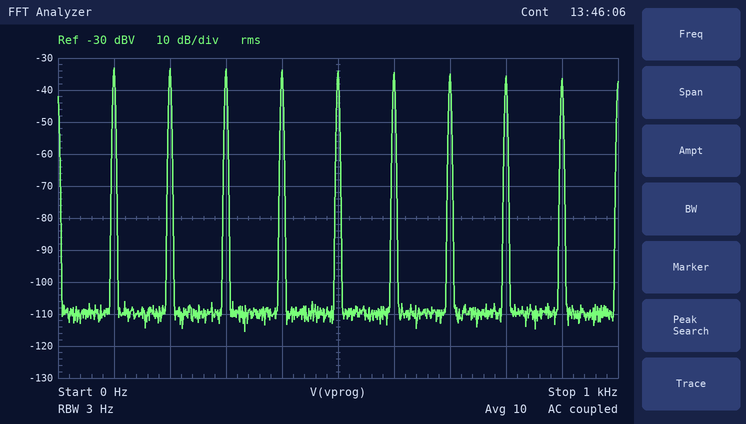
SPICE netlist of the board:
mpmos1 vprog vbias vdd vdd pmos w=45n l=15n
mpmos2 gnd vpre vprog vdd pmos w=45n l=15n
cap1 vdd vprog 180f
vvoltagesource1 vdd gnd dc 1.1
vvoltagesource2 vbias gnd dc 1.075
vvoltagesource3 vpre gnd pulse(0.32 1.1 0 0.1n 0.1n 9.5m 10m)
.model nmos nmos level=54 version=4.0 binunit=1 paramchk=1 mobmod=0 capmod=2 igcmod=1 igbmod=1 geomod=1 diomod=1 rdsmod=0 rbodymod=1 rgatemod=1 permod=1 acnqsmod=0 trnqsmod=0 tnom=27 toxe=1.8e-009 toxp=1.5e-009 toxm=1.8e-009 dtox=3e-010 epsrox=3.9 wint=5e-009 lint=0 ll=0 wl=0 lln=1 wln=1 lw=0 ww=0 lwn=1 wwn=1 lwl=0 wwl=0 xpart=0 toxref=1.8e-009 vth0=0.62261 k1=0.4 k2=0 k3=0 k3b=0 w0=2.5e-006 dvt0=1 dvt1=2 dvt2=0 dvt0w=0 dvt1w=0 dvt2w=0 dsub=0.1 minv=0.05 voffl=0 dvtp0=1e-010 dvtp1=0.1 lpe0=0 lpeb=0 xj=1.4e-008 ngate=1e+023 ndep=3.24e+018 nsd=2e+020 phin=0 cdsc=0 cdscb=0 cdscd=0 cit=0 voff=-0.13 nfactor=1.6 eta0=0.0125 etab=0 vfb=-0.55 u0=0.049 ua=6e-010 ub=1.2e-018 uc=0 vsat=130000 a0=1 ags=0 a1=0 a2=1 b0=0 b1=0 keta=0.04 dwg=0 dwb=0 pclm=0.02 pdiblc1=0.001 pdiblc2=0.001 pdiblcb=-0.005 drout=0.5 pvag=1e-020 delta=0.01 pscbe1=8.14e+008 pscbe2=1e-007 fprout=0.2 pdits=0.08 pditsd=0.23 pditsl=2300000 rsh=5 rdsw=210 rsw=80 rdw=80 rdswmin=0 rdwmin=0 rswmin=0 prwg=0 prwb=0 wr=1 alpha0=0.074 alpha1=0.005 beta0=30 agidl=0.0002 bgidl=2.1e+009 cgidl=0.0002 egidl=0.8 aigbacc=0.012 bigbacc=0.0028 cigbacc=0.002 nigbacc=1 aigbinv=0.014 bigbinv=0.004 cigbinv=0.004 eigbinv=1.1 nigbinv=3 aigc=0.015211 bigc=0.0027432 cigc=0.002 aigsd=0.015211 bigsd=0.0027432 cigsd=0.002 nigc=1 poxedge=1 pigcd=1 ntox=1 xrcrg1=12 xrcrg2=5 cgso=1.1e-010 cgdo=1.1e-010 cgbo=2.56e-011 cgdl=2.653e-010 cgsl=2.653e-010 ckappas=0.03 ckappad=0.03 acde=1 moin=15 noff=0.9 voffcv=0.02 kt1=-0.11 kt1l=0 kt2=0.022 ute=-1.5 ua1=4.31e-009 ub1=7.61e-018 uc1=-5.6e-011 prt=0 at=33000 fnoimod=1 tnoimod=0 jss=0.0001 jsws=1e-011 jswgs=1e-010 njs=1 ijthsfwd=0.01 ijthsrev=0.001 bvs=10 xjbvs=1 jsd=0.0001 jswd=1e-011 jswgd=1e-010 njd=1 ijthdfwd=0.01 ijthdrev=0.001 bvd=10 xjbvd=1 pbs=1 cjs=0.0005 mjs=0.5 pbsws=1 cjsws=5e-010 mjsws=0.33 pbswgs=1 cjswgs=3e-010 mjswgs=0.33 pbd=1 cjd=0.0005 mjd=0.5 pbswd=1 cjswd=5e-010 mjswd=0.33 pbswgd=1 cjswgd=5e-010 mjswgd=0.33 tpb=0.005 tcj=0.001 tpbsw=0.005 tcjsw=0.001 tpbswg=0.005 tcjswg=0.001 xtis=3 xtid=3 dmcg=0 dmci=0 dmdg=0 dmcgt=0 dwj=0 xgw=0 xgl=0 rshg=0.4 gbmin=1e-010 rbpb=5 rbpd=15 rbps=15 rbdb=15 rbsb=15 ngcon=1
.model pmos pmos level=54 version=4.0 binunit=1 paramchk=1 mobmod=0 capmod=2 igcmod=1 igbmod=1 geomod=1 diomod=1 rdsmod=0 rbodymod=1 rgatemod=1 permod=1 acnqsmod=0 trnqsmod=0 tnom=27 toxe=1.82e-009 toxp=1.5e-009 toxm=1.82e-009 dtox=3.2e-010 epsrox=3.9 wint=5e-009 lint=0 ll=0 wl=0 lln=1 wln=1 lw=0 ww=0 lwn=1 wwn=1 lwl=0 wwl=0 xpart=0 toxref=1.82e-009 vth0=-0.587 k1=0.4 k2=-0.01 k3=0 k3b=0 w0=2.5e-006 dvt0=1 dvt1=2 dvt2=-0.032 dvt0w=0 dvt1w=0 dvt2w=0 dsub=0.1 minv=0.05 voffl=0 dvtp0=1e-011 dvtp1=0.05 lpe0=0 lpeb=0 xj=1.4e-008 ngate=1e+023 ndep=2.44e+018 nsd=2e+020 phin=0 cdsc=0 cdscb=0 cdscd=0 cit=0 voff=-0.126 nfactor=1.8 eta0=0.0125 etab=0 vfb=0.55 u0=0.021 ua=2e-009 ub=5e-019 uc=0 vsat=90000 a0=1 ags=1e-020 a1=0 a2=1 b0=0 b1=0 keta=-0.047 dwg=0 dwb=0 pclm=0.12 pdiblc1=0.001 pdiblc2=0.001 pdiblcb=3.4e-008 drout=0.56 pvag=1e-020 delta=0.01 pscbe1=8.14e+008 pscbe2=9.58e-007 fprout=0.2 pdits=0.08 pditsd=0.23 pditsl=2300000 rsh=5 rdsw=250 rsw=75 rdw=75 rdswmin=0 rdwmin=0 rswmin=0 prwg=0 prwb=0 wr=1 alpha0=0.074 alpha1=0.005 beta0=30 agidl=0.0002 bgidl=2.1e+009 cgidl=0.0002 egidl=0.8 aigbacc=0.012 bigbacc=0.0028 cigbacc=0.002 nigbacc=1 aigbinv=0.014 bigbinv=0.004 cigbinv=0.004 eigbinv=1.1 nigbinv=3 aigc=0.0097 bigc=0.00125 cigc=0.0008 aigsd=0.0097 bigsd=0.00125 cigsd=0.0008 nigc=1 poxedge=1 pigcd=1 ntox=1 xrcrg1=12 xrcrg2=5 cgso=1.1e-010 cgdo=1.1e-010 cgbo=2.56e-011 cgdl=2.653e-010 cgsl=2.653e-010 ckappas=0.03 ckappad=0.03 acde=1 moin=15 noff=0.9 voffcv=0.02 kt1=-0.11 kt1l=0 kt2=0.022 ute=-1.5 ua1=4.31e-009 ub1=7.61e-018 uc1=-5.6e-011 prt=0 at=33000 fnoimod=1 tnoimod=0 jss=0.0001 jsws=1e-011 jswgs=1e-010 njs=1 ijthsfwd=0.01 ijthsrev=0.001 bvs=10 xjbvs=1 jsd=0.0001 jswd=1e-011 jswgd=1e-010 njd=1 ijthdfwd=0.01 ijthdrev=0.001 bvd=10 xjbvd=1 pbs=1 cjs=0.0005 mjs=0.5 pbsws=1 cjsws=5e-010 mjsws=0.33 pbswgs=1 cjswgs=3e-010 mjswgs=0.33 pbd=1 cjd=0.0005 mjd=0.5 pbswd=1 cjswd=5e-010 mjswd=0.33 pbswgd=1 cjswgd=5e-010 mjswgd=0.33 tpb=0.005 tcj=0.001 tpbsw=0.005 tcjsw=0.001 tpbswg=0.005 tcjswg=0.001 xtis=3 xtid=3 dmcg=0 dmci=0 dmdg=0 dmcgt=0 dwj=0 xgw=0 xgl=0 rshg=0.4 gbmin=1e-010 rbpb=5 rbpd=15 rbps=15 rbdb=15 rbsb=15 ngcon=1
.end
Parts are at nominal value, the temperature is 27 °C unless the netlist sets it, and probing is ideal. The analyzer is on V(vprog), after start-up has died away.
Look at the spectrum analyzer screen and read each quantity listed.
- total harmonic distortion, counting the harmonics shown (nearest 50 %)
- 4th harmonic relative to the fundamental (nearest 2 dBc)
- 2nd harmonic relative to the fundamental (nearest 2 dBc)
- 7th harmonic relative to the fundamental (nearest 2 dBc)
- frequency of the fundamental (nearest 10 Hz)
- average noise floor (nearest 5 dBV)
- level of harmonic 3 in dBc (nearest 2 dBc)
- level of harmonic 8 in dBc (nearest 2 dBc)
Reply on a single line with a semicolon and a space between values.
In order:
250 %; 0 dBc; 0 dBc; -2 dBc; 100 Hz; -110 dBV; 0 dBc; -2 dBc
